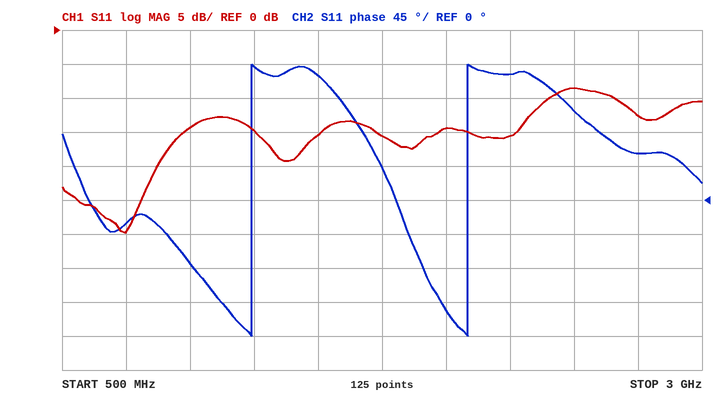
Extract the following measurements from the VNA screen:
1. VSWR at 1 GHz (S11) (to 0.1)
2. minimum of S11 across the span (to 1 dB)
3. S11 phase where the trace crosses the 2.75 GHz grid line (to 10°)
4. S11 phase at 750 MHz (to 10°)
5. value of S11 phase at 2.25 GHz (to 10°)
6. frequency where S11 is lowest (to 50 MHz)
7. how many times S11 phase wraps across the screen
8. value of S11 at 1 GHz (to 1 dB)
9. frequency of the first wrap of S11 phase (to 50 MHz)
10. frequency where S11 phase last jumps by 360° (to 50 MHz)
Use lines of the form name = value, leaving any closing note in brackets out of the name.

VSWR at 1 GHz (S11) = 1.5
minimum of S11 across the span = -30 dB
S11 phase where the trace crosses the 2.75 GHz grid line = 60°
S11 phase at 750 MHz = -30°
value of S11 phase at 2.25 GHz = 170°
frequency where S11 is lowest = 750 MHz
how many times S11 phase wraps across the screen = 2
value of S11 at 1 GHz = -14 dB
frequency of the first wrap of S11 phase = 1.25 GHz
frequency where S11 phase last jumps by 360° = 2.10 GHz
